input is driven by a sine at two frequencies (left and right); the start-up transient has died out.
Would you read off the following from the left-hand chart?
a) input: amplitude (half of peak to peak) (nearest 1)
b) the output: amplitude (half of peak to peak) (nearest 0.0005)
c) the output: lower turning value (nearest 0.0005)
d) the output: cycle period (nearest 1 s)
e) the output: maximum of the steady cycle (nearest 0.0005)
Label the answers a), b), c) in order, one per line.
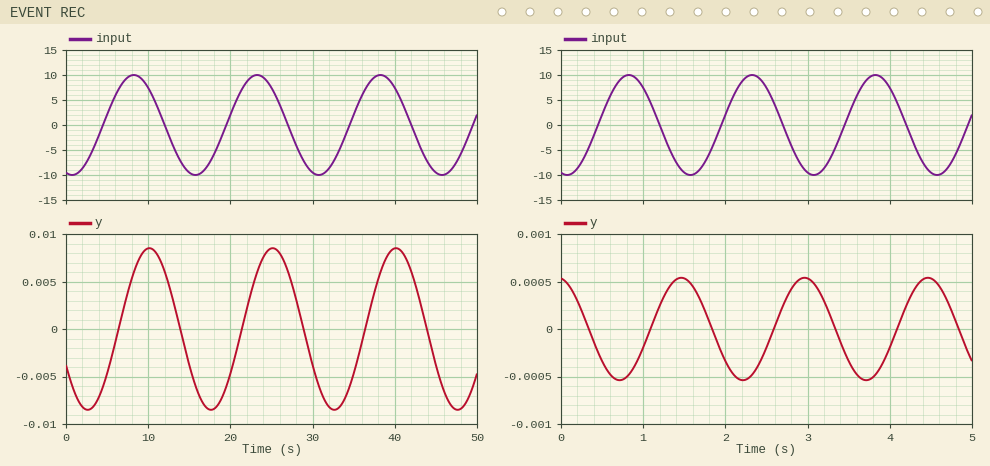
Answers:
a) 10
b) 0.0085
c) -0.0085
d) 15 s
e) 0.0085
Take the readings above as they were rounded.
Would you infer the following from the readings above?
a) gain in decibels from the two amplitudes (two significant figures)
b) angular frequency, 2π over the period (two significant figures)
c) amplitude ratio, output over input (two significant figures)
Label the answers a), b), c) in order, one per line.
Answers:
a) -61 dB
b) 0.42 rad/s
c) 0.00085
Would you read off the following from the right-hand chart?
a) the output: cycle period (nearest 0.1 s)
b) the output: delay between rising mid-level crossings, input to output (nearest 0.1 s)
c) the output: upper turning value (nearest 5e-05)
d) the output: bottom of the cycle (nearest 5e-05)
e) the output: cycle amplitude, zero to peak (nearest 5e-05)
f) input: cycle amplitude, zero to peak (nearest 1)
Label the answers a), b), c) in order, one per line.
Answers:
a) 1.5 s
b) 0.6 s
c) 0.00055
d) -0.00055
e) 0.00055
f) 10
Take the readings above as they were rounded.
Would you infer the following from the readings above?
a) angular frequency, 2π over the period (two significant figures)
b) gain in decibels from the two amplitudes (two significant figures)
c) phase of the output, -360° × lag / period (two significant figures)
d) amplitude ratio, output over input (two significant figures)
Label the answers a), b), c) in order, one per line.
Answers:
a) 4.2 rad/s
b) -85 dB
c) -140°
d) 0.000055
